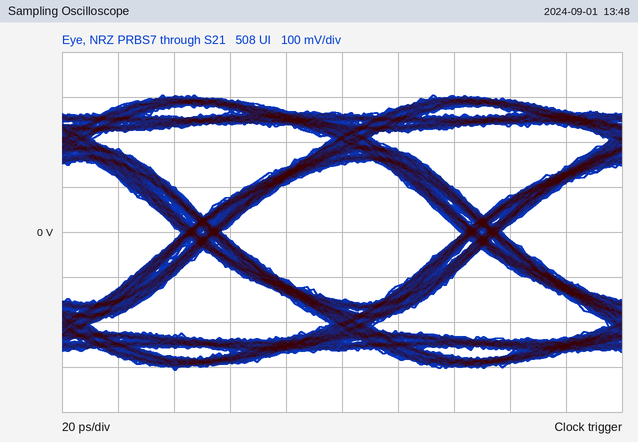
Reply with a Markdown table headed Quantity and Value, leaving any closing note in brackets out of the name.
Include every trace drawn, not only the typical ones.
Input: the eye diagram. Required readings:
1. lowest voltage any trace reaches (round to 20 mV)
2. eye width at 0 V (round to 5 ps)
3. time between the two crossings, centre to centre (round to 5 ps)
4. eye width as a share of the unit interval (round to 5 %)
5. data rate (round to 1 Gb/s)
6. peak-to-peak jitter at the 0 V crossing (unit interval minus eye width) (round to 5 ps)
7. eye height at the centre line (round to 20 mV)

| Quantity | Value |
|---|---|
| lowest voltage any trace reaches | -300 mV |
| eye width at 0 V | 85 ps |
| time between the two crossings, centre to centre | 100 ps |
| eye width as a share of the unit interval | 85 % |
| data rate | 10 Gb/s |
| peak-to-peak jitter at the 0 V crossing (unit interval minus eye width) | 15 ps |
| eye height at the centre line | 300 mV |
